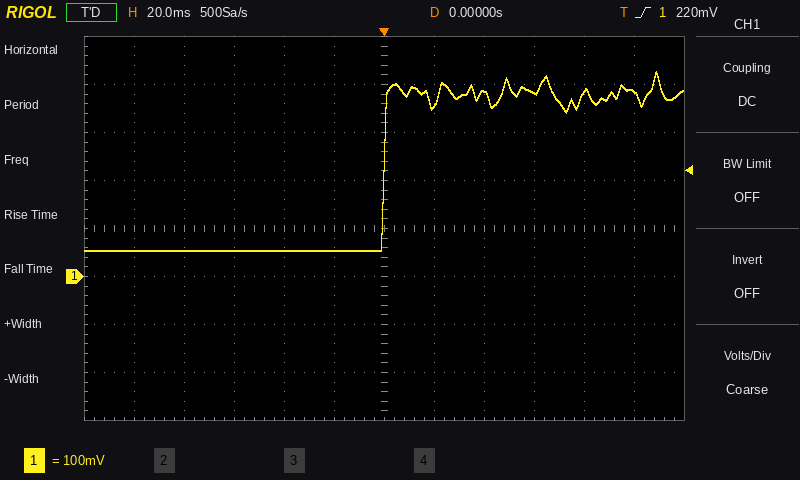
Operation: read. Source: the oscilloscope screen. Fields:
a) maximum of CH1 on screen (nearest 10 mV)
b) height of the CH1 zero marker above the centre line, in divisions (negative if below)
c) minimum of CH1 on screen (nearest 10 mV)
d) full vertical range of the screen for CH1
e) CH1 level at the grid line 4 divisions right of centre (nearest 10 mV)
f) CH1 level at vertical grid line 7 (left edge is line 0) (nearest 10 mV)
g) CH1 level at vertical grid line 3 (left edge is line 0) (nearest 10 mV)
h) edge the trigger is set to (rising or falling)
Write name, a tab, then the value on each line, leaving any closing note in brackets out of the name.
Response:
maximum of CH1 on screen	430 mV
height of the CH1 zero marker above the centre line, in divisions	-1.0 div
minimum of CH1 on screen	50 mV
full vertical range of the screen for CH1	800 mV
CH1 level at the grid line 4 divisions right of centre	380 mV
CH1 level at vertical grid line 7 (left edge is line 0)	360 mV
CH1 level at vertical grid line 3 (left edge is line 0)	50 mV
edge the trigger is set to	rising
